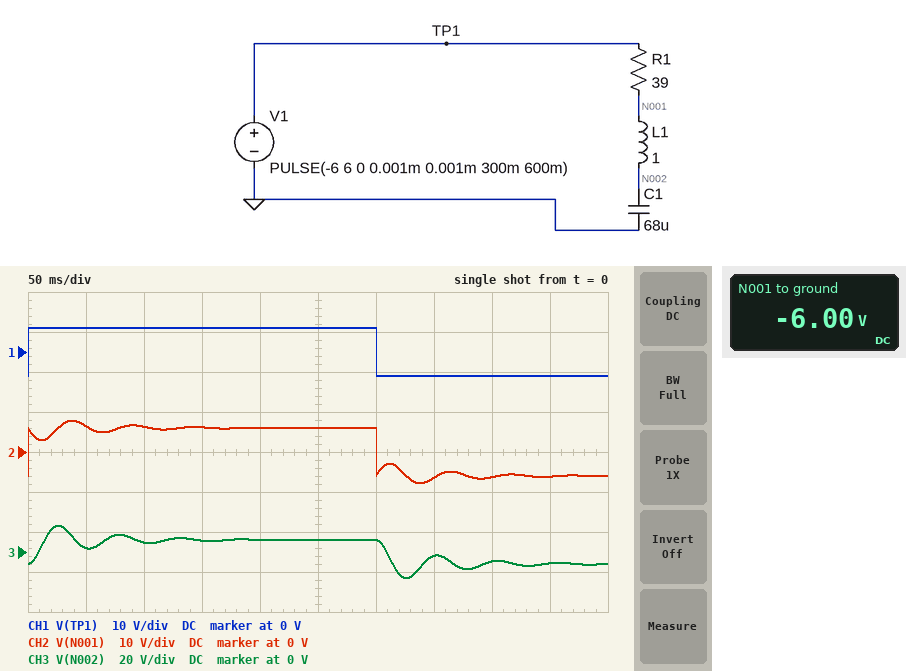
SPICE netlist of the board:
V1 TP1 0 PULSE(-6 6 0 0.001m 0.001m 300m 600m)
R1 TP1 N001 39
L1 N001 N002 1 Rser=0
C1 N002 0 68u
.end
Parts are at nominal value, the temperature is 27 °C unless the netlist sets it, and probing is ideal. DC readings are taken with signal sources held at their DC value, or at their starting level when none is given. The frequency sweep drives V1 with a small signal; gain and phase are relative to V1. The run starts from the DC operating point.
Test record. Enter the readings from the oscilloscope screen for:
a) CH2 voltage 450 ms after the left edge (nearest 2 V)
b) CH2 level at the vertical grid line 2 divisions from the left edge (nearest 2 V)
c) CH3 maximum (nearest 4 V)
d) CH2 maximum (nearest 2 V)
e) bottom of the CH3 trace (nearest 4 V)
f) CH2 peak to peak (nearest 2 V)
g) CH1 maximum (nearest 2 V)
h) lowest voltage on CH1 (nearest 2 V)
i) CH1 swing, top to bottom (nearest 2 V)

-6 V
6 V
12 V
8 V
-12 V
16 V
6 V
-6 V
12 V
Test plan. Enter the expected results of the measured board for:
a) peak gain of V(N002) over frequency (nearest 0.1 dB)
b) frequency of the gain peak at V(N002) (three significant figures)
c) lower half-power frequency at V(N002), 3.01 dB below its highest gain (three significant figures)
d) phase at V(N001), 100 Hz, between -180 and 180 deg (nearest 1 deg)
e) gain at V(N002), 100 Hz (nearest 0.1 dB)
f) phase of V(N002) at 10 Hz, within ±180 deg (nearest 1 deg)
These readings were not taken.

10.0 dB
18.8 Hz
15.3 Hz
4 deg
-28.3 dB
-13 deg
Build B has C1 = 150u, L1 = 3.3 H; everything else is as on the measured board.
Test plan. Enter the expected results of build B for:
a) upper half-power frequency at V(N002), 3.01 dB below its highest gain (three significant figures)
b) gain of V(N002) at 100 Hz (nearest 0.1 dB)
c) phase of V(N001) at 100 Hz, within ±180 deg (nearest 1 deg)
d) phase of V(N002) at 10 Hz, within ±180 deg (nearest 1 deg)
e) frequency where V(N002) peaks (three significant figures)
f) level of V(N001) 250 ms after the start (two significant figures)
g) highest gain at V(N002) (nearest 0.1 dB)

7.92 Hz
-45.8 dB
1 deg
-159 deg
7.03 Hz
6.7 V
11.7 dB
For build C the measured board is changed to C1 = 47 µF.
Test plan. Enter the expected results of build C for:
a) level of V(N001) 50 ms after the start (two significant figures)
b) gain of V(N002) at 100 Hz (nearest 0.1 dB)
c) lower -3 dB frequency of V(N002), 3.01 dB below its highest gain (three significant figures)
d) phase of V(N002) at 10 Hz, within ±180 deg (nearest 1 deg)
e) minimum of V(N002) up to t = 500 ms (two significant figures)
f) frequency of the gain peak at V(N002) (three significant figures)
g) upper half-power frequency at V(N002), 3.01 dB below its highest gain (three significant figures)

5.0 V
-24.9 dB
19.4 Hz
-8 deg
-14 V
22.8 Hz
25.7 Hz
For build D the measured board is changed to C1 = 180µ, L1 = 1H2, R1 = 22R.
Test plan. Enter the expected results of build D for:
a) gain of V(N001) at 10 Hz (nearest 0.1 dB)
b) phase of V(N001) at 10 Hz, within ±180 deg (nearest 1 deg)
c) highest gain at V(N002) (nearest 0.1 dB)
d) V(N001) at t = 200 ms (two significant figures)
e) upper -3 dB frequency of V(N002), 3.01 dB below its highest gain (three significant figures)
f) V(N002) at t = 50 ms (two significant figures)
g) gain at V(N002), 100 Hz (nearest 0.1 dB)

-5.9 dB
-59 deg
11.5 dB
5.6 V
12.0 Hz
14 V
-38.5 dB
